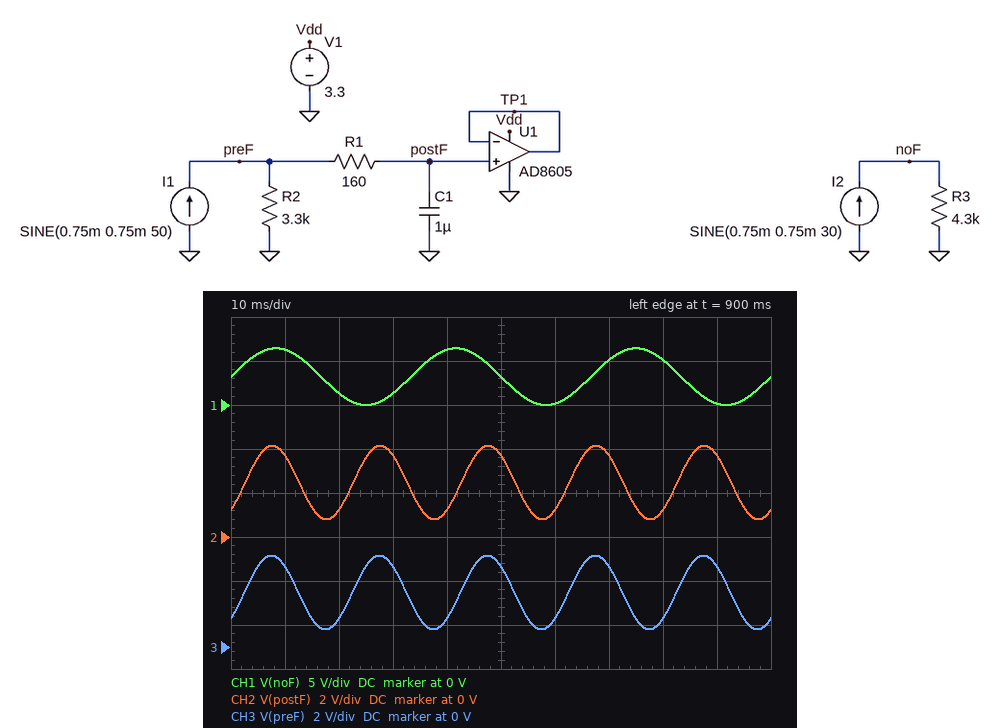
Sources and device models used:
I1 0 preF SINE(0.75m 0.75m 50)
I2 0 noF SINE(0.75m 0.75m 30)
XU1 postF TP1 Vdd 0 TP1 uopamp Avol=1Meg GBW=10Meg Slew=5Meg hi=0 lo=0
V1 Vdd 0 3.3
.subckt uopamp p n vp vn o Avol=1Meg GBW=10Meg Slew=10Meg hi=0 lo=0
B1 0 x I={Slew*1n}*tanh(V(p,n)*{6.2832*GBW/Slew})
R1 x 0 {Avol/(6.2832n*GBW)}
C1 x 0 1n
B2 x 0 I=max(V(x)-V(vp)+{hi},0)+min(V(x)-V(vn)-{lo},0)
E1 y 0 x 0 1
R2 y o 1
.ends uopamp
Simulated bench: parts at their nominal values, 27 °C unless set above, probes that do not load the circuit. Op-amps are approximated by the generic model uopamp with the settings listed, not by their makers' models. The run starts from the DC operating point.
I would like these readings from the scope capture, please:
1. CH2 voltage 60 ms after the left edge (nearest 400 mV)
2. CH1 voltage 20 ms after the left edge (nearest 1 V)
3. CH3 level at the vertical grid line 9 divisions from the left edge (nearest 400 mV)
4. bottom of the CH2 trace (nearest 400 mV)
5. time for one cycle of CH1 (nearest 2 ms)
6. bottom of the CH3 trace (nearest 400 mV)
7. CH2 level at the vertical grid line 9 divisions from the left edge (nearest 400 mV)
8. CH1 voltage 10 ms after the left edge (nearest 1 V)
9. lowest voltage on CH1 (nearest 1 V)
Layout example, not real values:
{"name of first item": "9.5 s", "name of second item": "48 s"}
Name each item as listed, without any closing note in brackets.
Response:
{"CH2 voltage 60 ms after the left edge": "1.2 V", "CH1 voltage 20 ms after the left edge": "1 V", "CH3 level at the vertical grid line 9 divisions from the left edge": "3.6 V", "bottom of the CH2 trace": "800 mV", "time for one cycle of CH1": "34 ms", "bottom of the CH3 trace": "800 mV", "CH2 level at the vertical grid line 9 divisions from the left edge": "3.6 V", "CH1 voltage 10 ms after the left edge": "6 V", "lowest voltage on CH1": "0 V"}
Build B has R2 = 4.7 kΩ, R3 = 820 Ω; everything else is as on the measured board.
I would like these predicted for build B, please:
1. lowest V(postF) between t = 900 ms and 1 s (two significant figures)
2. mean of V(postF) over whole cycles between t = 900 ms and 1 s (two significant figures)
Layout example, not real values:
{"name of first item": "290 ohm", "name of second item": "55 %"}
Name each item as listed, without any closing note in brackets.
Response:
{"lowest V(postF) between t = 900 ms and 1 s": "1.6 V", "mean of V(postF) over whole cycles between t = 900 ms and 1 s": "3.5 V"}
